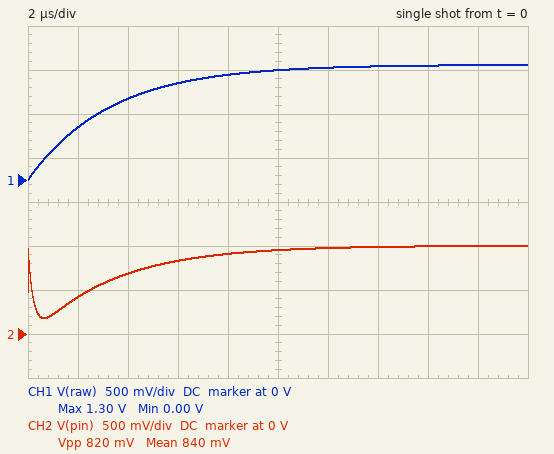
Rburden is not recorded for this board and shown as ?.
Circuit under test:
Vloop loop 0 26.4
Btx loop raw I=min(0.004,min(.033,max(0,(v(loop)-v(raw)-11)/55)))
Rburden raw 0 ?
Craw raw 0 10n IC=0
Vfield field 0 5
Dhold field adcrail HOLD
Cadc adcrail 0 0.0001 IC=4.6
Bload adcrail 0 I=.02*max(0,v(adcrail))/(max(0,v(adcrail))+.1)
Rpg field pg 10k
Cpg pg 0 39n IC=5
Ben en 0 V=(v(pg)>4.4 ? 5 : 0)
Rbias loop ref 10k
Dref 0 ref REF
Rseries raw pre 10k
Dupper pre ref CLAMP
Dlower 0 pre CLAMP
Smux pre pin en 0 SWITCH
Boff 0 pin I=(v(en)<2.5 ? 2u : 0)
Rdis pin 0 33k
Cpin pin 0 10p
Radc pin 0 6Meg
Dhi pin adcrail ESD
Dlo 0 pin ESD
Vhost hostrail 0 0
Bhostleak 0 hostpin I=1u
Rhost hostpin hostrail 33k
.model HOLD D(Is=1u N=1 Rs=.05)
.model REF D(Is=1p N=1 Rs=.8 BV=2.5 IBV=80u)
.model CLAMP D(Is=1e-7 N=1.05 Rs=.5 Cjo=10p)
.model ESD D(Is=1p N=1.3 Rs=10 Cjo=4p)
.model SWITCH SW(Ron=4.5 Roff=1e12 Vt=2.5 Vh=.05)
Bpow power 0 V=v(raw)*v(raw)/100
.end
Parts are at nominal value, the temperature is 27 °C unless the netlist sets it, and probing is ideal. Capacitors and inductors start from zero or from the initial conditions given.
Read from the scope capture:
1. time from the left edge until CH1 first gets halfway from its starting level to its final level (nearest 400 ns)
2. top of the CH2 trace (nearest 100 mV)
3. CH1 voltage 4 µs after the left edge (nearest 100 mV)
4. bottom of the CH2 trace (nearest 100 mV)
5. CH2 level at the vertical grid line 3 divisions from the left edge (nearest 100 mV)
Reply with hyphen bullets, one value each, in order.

- 2.4 µs
- 1.0 V
- 900 mV
- 200 mV
- 800 mV
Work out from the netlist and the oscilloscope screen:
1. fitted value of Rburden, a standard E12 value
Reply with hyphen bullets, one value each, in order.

- 330 Ω
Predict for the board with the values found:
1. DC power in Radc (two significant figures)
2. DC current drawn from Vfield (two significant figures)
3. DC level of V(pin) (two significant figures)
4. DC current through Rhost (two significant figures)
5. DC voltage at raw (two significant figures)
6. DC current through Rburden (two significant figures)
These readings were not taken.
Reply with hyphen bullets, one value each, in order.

- 170 nW
- 20 mA
- 1.0 V
- 1.0 µA
- 1.3 V
- 4.0 mA
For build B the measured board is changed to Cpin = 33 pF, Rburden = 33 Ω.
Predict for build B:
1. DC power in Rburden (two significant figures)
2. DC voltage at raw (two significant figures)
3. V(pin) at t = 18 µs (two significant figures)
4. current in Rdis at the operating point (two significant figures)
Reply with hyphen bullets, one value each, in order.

- 530 µW
- 130 mV
- 100 mV
- 3.1 µA
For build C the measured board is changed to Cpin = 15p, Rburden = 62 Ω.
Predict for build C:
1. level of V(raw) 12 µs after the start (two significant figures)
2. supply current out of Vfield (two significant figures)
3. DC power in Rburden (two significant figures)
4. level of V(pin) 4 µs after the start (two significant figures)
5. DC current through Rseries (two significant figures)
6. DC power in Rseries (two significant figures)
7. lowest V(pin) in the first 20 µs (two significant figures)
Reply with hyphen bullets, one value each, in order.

- 250 mV
- 20 mA
- 990 µW
- 190 mV
- 5.8 µA
- 330 nW
- 150 mV
